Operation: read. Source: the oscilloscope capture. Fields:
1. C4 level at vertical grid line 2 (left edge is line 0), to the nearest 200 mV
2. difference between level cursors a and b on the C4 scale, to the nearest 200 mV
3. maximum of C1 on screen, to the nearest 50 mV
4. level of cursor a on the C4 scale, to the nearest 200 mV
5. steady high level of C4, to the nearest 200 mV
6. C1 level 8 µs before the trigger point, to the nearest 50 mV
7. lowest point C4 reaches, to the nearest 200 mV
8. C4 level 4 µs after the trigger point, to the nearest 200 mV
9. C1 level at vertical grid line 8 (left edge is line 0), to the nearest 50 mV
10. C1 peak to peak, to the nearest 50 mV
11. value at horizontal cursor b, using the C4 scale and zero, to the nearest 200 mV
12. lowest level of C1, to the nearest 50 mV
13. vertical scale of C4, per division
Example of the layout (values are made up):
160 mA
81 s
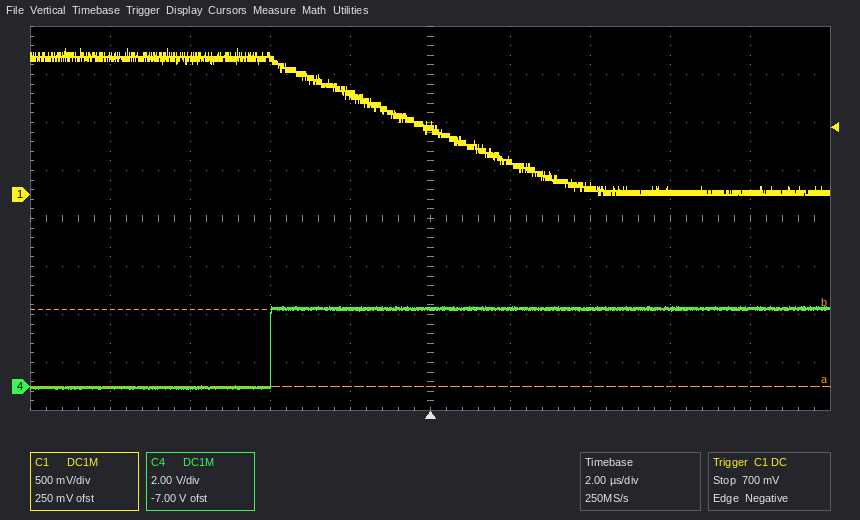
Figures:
0.0 V
3.2 V
1.50 V
0.0 V
3.2 V
1.45 V
-200 mV
3.2 V
50 mV
1.50 V
3.2 V
0 mV
2 V
